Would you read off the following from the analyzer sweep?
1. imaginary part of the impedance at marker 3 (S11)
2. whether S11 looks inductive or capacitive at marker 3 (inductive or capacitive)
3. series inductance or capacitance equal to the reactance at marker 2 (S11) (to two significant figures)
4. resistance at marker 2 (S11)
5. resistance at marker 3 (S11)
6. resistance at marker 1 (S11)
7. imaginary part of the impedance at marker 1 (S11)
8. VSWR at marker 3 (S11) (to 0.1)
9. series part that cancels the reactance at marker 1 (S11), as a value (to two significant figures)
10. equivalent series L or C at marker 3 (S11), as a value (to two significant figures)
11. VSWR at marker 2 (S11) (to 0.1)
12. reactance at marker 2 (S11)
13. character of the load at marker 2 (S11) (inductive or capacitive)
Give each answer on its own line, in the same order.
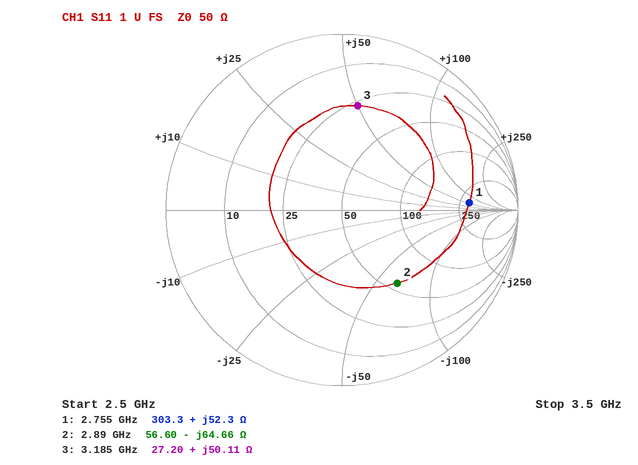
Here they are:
+50.11 Ω
inductive
850 fF
56.60 Ω
27.20 Ω
303.3 Ω
+52.3 Ω
4.0
1.1 pF
2.5 nH
3.2
-64.66 Ω
capacitive
